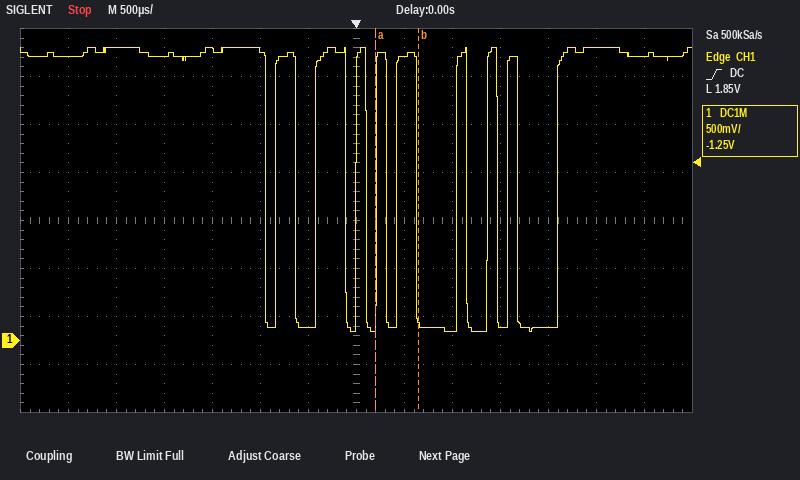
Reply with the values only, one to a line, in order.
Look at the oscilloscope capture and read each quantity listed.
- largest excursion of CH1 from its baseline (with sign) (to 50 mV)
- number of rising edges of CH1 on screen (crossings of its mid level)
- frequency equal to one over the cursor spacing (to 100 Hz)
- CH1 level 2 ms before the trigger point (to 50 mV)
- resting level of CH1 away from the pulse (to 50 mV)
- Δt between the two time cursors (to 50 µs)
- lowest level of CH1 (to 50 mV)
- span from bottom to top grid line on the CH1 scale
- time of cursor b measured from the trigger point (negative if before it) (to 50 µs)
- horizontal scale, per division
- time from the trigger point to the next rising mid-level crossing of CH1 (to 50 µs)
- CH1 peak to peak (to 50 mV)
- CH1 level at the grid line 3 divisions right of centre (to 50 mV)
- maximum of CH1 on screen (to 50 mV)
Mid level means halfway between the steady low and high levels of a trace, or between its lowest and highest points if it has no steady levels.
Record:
-2.85 V
9
2.2 kHz
2.95 V
2.95 V
450 µs
100 mV
4 V
+650 µs
500 µs
200 µs
2.95 V
150 mV
3.05 V
